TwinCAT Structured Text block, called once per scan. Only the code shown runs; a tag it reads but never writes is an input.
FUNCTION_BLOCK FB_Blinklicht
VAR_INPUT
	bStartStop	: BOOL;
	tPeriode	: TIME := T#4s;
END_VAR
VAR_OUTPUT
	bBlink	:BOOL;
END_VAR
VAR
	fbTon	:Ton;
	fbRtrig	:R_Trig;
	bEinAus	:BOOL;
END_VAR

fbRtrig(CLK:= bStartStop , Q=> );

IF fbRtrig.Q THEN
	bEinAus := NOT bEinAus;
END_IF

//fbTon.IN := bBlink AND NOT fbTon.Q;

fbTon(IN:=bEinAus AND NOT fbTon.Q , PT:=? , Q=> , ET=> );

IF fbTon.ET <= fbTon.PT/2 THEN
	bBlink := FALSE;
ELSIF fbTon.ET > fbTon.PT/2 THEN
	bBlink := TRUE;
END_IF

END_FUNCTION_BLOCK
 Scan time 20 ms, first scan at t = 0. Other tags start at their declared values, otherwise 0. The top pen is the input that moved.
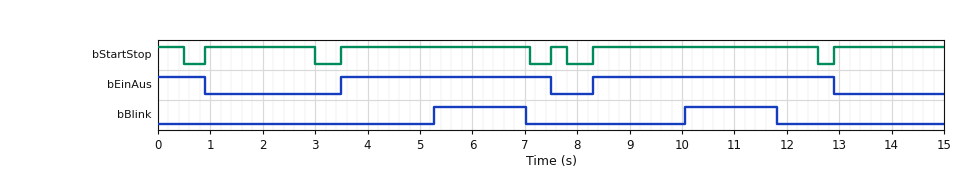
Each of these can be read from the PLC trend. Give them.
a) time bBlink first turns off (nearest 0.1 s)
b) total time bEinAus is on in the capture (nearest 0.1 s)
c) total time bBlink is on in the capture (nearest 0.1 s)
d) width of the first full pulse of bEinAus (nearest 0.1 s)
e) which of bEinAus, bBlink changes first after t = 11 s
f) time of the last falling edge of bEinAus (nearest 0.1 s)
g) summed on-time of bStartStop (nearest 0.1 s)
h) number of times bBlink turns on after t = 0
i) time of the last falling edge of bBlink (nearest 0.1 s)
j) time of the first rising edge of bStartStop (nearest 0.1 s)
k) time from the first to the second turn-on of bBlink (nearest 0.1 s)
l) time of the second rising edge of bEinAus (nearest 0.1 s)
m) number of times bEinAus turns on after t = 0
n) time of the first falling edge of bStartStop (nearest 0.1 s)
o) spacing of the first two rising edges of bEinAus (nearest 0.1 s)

7.0 s
9.5 s
3.5 s
4.0 s
bBlink
12.9 s
12.9 s
2
11.8 s
0.9 s
4.8 s
8.3 s
2
0.5 s
4.8 s
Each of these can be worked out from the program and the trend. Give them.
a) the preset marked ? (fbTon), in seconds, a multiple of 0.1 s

3.5 s
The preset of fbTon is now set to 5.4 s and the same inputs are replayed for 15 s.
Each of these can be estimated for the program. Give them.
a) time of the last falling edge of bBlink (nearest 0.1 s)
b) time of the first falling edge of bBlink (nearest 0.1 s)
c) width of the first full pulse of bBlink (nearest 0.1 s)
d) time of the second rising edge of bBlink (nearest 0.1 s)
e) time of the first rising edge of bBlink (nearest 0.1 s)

12.9 s
7.5 s
1.3 s
11.0 s
6.2 s
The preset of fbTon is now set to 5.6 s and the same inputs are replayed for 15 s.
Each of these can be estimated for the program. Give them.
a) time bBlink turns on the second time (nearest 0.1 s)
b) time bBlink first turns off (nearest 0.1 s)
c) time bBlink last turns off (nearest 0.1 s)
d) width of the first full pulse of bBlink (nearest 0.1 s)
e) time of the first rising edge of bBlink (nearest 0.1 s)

11.1 s
7.5 s
12.9 s
1.2 s
6.3 s
